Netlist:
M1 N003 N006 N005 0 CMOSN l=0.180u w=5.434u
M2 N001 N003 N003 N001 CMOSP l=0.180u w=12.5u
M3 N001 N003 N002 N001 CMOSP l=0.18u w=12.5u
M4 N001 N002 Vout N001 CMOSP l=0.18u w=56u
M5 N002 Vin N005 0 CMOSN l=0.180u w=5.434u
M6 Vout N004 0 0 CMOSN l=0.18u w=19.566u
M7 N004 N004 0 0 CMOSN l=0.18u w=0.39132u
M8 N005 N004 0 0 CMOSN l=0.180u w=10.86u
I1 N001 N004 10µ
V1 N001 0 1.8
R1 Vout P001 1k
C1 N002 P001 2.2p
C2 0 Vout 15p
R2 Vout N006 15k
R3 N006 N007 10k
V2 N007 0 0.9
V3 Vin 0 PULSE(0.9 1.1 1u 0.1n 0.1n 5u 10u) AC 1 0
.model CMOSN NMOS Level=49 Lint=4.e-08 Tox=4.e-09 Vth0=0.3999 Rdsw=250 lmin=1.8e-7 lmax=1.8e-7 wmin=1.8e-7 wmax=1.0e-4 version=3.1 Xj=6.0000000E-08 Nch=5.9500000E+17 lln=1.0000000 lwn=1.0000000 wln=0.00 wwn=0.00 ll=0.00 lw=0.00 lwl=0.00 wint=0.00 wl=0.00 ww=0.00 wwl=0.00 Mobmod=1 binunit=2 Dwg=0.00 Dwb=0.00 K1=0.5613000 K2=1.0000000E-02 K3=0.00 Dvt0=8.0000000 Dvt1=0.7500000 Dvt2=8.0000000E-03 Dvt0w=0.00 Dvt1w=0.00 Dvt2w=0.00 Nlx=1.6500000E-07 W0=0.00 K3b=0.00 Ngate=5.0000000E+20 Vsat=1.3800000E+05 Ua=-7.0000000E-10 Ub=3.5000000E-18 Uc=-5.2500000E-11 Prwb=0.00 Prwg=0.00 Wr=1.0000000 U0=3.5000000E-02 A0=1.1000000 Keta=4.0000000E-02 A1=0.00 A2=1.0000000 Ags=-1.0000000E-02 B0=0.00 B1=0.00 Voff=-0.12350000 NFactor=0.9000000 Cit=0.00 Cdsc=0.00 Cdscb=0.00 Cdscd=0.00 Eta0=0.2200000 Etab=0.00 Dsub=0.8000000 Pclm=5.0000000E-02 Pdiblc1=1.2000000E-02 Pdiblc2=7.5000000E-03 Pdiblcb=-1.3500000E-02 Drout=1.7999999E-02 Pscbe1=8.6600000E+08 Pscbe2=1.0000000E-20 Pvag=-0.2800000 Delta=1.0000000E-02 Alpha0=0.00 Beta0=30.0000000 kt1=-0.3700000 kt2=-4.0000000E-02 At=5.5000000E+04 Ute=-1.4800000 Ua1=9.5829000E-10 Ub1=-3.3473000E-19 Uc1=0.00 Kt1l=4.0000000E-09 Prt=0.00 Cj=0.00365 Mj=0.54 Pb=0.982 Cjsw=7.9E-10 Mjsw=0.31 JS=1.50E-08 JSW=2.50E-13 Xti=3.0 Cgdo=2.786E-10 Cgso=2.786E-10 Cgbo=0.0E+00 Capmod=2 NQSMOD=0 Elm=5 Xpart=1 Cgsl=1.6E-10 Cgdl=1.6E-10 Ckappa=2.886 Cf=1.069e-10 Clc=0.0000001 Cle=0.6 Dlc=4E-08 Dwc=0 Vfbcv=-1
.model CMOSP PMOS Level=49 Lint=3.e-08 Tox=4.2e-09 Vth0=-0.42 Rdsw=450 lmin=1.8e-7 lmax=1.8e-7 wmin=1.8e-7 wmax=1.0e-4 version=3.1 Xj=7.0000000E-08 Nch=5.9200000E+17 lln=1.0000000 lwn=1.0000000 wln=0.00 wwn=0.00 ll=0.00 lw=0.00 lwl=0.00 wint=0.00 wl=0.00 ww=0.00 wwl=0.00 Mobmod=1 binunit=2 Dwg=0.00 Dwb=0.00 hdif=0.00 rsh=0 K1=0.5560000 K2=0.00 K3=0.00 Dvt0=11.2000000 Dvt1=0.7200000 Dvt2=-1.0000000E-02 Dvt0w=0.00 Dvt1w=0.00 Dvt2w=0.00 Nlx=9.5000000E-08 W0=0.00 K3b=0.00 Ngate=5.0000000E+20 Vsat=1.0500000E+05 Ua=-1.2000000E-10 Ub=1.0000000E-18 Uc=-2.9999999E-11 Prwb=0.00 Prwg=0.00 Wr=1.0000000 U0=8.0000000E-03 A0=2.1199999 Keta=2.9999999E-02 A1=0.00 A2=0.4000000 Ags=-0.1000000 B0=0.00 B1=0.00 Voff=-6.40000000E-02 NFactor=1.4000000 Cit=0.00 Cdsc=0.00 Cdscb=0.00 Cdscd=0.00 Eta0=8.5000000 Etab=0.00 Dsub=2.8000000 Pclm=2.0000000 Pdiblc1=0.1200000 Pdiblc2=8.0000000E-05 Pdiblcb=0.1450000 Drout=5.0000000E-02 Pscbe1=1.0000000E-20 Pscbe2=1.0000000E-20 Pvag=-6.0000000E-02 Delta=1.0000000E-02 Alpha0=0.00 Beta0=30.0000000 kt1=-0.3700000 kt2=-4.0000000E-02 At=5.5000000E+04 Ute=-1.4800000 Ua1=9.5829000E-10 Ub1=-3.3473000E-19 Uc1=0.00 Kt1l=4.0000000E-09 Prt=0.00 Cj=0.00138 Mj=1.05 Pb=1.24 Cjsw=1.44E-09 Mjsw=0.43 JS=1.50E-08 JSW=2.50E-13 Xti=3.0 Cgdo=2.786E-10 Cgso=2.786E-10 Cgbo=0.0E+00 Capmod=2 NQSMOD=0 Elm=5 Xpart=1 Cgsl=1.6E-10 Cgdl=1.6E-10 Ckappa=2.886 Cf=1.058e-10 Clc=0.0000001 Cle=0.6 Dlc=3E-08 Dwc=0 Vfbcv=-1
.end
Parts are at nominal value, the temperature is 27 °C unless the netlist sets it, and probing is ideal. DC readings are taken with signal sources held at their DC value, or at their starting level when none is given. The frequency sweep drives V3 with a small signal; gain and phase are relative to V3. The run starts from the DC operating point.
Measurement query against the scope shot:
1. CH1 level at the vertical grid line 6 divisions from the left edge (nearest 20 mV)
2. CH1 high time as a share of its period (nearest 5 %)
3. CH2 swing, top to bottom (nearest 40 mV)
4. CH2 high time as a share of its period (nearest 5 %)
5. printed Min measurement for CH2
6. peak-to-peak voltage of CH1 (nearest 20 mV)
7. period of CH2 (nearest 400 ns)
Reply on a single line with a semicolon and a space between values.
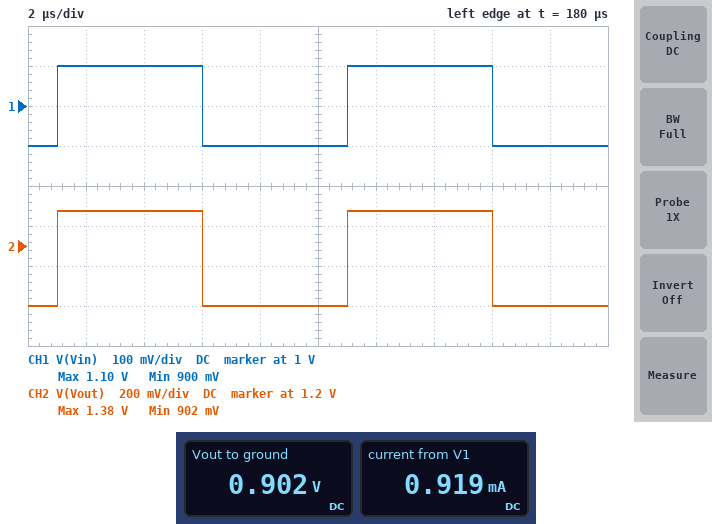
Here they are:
1.10 V; 50 %; 480 mV; 50 %; 902 mV; 200 mV; 10.0 µs
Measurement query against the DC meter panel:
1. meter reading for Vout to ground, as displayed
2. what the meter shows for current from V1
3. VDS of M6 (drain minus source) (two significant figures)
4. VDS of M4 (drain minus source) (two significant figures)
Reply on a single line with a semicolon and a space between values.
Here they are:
0.902 V; 0.919 mA; 900 mV; 900 mV
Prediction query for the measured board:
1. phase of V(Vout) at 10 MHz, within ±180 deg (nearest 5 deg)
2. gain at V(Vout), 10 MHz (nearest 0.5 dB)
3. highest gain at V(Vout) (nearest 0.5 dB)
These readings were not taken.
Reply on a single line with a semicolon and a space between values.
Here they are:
-20 deg; 7.0 dB; 7.5 dB
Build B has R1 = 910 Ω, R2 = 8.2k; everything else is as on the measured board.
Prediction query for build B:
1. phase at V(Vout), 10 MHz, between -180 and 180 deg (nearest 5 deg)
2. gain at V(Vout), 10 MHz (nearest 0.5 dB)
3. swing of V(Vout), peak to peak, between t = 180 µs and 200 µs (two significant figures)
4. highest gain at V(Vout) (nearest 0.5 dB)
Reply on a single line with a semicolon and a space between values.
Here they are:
-15 deg; 4.5 dB; 350 mV; 5.0 dB
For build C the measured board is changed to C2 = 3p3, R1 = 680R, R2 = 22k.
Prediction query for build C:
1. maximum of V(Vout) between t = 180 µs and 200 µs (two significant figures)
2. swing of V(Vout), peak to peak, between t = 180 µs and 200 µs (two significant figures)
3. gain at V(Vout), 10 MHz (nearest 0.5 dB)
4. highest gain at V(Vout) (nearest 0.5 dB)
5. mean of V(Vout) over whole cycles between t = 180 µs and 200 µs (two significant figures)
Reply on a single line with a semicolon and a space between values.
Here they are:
1.5 V; 590 mV; 9.0 dB; 9.5 dB; 1.2 V
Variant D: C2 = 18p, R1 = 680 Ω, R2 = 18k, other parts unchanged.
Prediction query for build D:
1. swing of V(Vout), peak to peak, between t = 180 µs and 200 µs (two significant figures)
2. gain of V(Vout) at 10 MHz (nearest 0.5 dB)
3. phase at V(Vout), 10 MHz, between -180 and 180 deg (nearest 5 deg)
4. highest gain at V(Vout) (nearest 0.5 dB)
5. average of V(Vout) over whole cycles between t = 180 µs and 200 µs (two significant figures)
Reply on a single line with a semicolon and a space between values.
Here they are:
530 mV; 8.0 dB; -25 deg; 8.5 dB; 1.2 V
